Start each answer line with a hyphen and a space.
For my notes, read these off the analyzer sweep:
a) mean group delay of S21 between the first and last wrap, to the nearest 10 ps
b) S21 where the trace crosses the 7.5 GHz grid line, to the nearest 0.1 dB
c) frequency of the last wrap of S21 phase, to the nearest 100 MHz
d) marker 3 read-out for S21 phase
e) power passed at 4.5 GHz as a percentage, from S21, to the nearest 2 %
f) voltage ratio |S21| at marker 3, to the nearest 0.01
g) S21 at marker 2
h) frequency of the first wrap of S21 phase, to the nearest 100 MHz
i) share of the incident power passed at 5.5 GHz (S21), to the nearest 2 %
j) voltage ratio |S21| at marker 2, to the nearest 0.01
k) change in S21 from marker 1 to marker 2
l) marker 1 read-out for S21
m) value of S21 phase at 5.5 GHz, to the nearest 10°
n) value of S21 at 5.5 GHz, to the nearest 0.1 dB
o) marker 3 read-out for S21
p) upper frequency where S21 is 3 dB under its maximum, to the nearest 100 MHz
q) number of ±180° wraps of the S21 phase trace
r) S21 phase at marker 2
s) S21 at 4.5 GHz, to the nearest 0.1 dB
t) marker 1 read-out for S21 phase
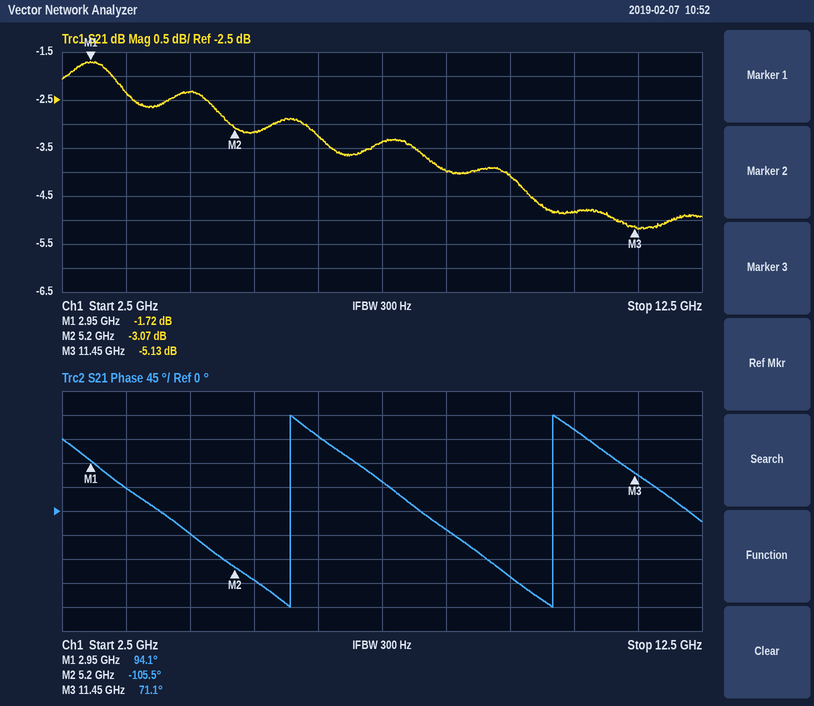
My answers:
- 240 ps
- -3.4 dB
- 10.2 GHz
- 71.1°
- 58 %
- 0.55
- -3.07 dB
- 6.1 GHz
- 48 %
- 0.70
- -1.35 dB
- -1.72 dB
- -130°
- -3.2 dB
- -5.13 dB
- 10.0 GHz
- 2
- -105.5°
- -2.3 dB
- 94.1°
